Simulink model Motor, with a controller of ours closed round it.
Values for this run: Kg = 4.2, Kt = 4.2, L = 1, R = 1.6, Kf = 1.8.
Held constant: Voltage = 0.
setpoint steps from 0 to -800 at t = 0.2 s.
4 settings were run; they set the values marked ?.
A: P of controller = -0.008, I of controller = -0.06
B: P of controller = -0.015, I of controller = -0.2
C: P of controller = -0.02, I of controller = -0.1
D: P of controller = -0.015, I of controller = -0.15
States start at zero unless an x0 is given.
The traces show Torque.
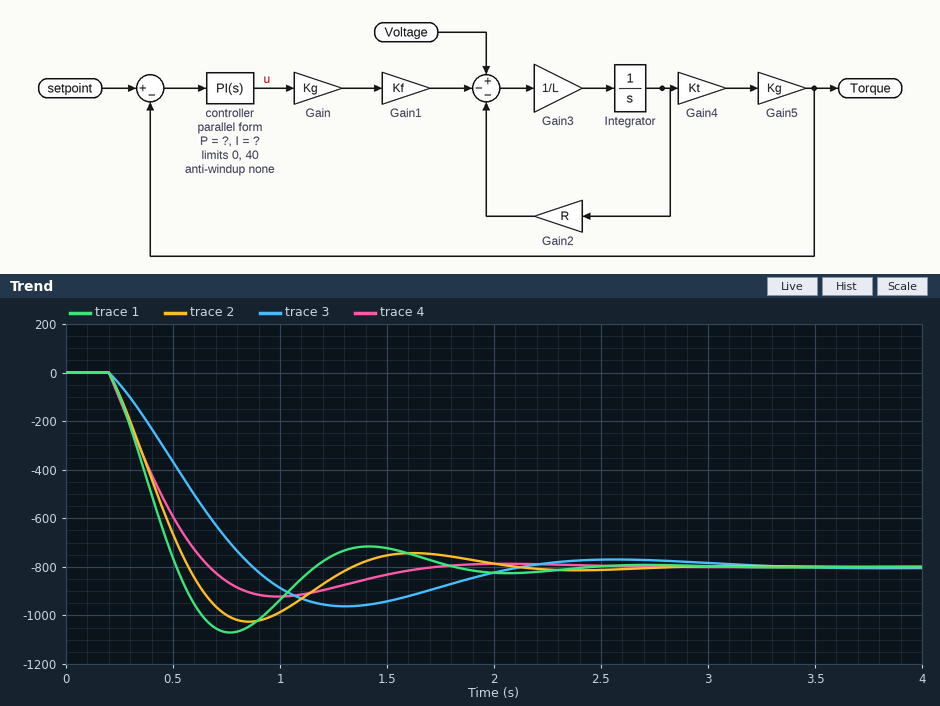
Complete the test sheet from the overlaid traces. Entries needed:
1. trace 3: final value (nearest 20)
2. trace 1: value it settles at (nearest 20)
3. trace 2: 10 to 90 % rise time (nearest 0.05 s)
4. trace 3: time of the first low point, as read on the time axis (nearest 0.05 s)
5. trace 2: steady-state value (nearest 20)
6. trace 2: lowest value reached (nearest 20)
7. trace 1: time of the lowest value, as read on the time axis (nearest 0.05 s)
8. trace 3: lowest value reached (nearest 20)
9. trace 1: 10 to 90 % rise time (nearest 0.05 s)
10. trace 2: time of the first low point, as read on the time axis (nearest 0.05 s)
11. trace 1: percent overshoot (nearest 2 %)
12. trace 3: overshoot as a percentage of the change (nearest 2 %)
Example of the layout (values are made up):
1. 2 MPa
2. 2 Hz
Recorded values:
1. -800
2. -800
3. 0.30 s
4. 1.30 s
5. -800
6. -1020
7. 0.75 s
8. -960
9. 0.25 s
10. 0.85 s
11. 34 %
12. 20 %
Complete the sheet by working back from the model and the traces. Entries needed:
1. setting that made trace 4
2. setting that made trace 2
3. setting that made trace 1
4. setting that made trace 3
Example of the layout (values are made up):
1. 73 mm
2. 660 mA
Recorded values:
1. C
2. D
3. B
4. A
